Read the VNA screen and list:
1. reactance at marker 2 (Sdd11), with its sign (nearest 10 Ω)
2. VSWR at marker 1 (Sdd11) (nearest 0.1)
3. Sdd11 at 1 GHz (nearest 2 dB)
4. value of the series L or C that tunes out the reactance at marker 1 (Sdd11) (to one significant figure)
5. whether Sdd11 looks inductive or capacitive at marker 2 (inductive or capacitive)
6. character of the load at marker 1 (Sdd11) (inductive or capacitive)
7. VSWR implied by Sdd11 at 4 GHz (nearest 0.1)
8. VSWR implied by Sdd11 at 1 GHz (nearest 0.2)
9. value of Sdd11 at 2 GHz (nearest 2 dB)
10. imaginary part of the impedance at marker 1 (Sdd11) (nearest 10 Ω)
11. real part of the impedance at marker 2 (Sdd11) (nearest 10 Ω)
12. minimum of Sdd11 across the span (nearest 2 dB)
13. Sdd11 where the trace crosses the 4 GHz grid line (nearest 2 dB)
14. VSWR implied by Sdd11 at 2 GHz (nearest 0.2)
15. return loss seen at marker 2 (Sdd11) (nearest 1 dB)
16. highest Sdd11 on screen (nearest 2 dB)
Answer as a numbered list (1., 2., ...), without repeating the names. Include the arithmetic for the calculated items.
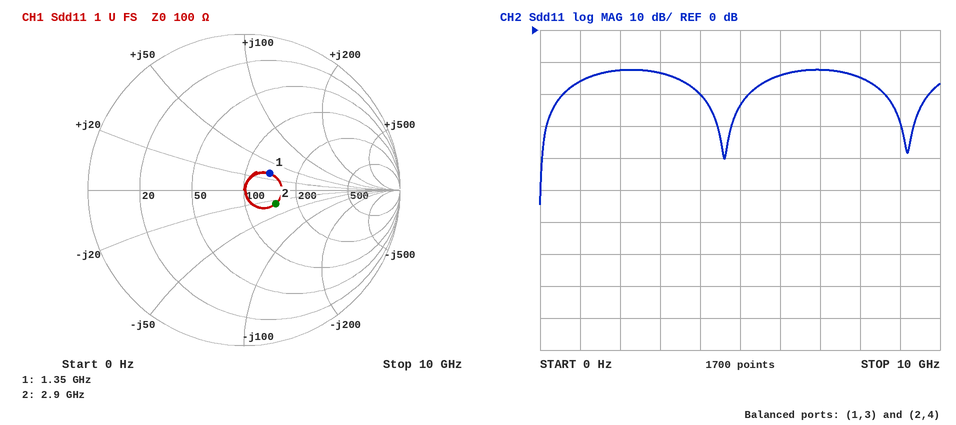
1. -30 Ω
2. 1.5
3. -16 dB
4. C = 1/(2π × 1.35 GHz × 30 Ω) ≈ 4 pF
5. capacitive
6. inductive
7. |Γ| = 10^(-20/20) = 0.1000; VSWR = (1 + 0.1000)/(1 − 0.1000) ≈ 1.2
8. |Γ| = 10^(-16/20) = 0.1585; VSWR = (1 + 0.1585)/(1 − 0.1585) ≈ 1.4
9. -12 dB
10. +30 Ω
11. 150 Ω
12. -54 dB
13. -20 dB
14. |Γ| = 10^(-12/20) = 0.2512; VSWR = (1 + 0.2512)/(1 − 0.2512) ≈ 1.67, so 1.6 to the nearest 0.2
15. 13 dB
16. -12 dB
